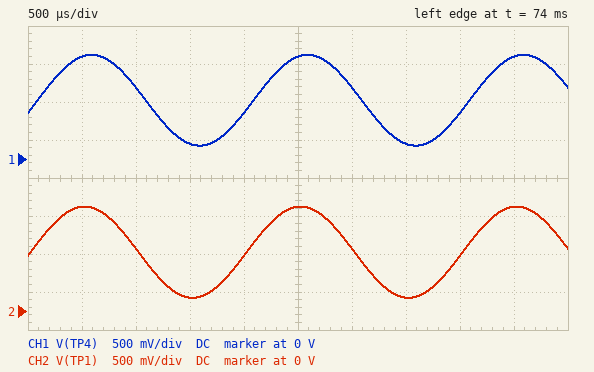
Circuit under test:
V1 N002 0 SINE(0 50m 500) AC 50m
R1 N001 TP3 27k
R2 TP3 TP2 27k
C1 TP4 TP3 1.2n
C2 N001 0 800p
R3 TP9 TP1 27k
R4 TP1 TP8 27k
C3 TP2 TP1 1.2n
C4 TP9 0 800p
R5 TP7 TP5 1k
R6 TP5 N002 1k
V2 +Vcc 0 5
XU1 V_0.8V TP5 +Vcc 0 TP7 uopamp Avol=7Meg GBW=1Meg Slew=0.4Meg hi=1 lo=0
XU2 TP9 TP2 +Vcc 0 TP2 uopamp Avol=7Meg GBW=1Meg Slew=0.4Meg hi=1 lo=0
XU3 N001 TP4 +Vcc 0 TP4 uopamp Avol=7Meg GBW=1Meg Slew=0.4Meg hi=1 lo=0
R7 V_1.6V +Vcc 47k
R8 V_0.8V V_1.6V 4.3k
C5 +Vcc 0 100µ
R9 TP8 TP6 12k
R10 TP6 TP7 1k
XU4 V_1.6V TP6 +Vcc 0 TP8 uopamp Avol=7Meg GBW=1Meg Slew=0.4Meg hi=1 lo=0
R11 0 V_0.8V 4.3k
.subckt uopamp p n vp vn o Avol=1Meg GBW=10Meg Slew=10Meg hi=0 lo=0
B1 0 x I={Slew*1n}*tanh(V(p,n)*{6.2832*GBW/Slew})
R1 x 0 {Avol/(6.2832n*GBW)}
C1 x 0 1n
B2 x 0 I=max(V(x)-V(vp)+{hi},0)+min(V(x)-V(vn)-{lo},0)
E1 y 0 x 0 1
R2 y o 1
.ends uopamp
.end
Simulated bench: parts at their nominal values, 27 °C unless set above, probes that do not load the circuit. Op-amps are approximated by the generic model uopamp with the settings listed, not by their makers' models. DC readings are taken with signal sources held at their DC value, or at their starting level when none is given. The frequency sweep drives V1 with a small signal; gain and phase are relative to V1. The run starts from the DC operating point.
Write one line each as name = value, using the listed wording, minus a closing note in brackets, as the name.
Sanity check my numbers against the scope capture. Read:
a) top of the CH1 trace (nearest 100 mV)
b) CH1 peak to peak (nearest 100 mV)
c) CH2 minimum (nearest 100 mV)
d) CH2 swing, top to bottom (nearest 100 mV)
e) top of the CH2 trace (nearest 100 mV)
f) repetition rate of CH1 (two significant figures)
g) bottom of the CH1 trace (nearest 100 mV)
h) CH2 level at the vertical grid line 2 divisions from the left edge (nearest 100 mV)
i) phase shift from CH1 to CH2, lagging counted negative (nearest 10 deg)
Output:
top of the CH1 trace = 1.4 V
CH1 peak to peak = 1.2 V
CH2 minimum = 200 mV
CH2 swing, top to bottom = 1.2 V
top of the CH2 trace = 1.4 V
repetition rate of CH1 = 500 Hz
bottom of the CH1 trace = 200 mV
CH2 level at the vertical grid line 2 divisions from the left edge = 800 mV
phase shift from CH1 to CH2, lagging counted negative = 10 deg
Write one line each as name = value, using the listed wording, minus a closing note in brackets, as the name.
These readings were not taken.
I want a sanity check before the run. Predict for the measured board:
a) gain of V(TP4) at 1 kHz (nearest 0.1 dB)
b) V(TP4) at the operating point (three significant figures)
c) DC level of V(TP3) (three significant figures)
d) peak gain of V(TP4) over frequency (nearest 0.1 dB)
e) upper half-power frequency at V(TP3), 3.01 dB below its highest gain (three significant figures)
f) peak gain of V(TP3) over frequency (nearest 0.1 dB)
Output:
gain of V(TP4) at 1 kHz = 21.4 dB
V(TP4) at the operating point = 773 mV
DC level of V(TP3) = 773 mV
peak gain of V(TP4) over frequency = 21.6 dB
upper half-power frequency at V(TP3), 3.01 dB below its highest gain = 4.42 kHz
peak gain of V(TP3) over frequency = 21.6 dB
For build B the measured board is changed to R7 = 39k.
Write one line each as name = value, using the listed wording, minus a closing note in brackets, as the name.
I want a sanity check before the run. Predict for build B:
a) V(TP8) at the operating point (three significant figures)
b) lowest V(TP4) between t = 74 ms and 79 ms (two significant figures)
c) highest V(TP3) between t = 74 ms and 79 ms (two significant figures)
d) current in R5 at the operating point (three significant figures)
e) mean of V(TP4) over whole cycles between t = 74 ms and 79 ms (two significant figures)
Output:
V(TP8) at the operating point = 903 mV
lowest V(TP4) between t = 74 ms and 79 ms = 310 mV
highest V(TP3) between t = 74 ms and 79 ms = 1.5 V
current in R5 at the operating point = 452 µA
mean of V(TP4) over whole cycles between t = 74 ms and 79 ms = 900 mV
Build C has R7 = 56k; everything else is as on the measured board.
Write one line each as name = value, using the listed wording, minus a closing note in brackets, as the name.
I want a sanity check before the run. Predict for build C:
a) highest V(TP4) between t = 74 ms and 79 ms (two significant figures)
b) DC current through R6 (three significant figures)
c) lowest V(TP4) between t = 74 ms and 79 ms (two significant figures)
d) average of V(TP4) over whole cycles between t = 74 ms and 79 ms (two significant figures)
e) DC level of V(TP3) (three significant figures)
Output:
highest V(TP4) between t = 74 ms and 79 ms = 1.3 V
DC current through R6 = 333 µA
lowest V(TP4) between t = 74 ms and 79 ms = 68 mV
average of V(TP4) over whole cycles between t = 74 ms and 79 ms = 670 mV
DC level of V(TP3) = 666 mV
